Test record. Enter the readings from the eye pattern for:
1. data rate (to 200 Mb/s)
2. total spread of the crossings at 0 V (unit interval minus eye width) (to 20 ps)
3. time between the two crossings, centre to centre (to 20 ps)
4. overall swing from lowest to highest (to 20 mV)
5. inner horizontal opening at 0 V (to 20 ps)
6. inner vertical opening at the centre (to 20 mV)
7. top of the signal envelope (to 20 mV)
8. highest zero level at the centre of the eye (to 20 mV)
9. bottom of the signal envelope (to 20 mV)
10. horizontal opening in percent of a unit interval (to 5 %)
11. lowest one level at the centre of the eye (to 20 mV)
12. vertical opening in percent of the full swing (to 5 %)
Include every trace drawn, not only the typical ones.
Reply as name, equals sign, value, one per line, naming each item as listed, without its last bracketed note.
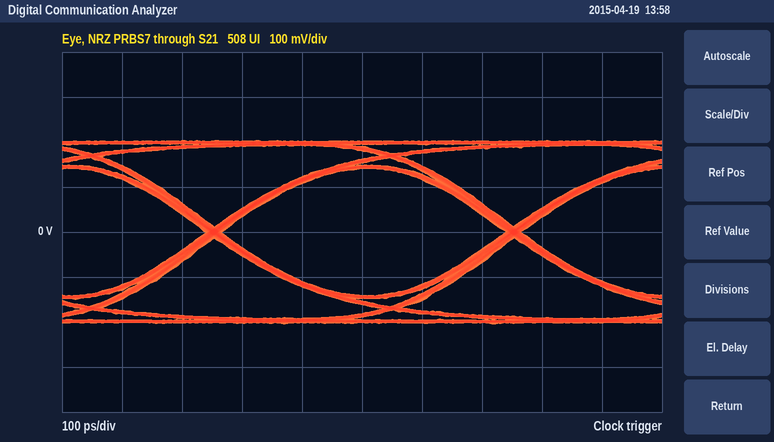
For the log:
data rate = 2.0 Gb/s
total spread of the crossings at 0 V (unit interval minus eye width) = 20 ps
time between the two crossings, centre to centre = 500 ps
overall swing from lowest to highest = 400 mV
inner horizontal opening at 0 V = 480 ps
inner vertical opening at the centre = 280 mV
top of the signal envelope = 200 mV
highest zero level at the centre of the eye = -140 mV
bottom of the signal envelope = -200 mV
horizontal opening in percent of a unit interval = 95 %
lowest one level at the centre of the eye = 140 mV
vertical opening in percent of the full swing = 70 %
